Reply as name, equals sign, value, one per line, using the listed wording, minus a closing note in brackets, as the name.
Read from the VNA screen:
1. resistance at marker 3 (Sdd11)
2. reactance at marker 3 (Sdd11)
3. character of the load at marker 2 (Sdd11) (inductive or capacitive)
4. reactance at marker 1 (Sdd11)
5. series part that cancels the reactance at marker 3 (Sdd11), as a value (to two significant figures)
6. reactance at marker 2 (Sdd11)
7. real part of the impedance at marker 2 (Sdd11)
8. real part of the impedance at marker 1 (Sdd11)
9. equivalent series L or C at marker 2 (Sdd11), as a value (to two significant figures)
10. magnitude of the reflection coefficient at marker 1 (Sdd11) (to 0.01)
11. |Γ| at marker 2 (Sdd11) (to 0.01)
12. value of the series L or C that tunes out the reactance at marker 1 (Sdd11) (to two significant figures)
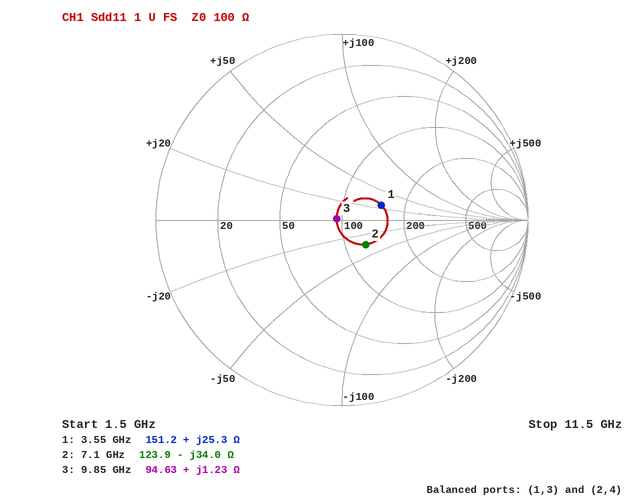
resistance at marker 3 = 94.63 Ω
reactance at marker 3 = +1.23 Ω
character of the load at marker 2 (Sdd11) = capacitive
reactance at marker 1 = +25.3 Ω
series part that cancels the reactance at marker 3 (Sdd11), as a value = 13 pF
reactance at marker 2 = -34.0 Ω
real part of the impedance at marker 2 = 123.9 Ω
real part of the impedance at marker 1 = 151.2 Ω
equivalent series L or C at marker 2 (Sdd11), as a value = 660 fF
magnitude of the reflection coefficient at marker 1 (Sdd11) = 0.23
|Γ| at marker 2 (Sdd11) = 0.18
value of the series L or C that tunes out the reactance at marker 1 (Sdd11) = 1.8 pF
